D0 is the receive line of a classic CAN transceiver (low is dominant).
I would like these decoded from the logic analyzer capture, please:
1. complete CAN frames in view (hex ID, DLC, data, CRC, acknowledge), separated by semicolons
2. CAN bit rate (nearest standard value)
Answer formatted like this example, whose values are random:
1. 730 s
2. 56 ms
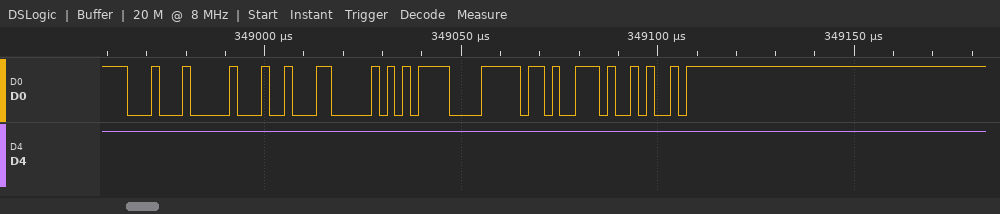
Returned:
1. ID 110, DLC 4, data 8C 0A F0 FE, CRC 4E94, ACK
2. 500 kbit/s
